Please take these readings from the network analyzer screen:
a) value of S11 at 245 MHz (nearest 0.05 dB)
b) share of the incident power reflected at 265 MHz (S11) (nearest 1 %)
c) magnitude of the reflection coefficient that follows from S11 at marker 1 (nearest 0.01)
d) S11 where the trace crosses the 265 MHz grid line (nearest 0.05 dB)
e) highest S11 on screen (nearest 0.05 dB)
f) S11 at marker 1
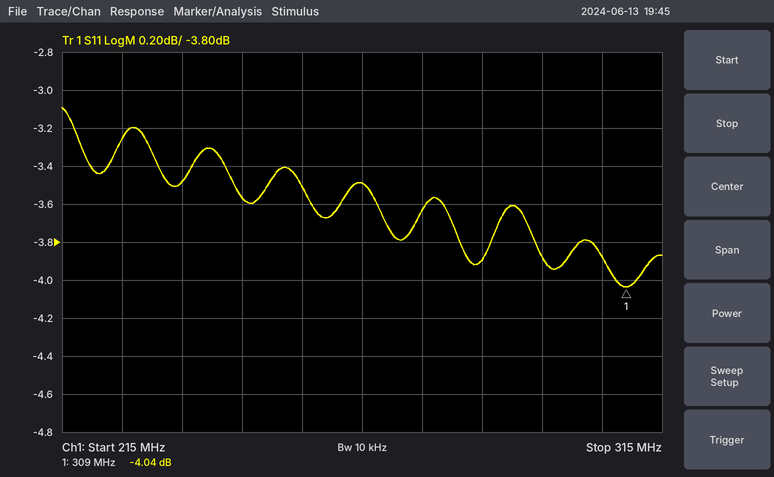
-3.55 dB
45 %
0.63
-3.50 dB
-3.10 dB
-4.04 dB
